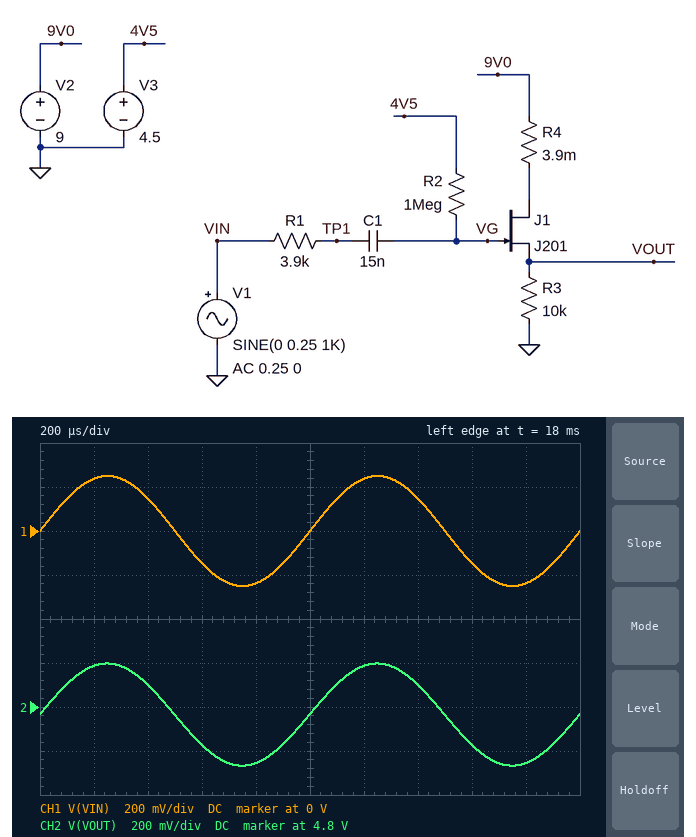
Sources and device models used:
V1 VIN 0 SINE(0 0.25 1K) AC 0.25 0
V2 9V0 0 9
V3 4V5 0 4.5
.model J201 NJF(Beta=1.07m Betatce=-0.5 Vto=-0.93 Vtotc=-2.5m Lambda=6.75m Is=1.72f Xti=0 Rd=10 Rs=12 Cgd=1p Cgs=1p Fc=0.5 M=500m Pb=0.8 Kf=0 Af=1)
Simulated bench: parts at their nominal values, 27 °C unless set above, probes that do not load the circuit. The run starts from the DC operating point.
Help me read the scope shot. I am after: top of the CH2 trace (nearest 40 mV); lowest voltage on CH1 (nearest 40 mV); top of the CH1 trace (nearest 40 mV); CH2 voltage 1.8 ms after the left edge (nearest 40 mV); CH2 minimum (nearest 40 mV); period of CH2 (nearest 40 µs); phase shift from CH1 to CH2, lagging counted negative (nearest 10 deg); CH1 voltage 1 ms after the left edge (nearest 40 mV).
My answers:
5.00 V
-240 mV
240 mV
4.56 V
4.52 V
1.00 ms
0 deg
0 V
